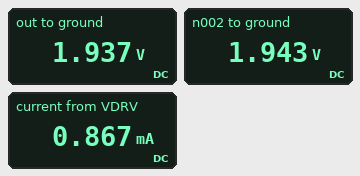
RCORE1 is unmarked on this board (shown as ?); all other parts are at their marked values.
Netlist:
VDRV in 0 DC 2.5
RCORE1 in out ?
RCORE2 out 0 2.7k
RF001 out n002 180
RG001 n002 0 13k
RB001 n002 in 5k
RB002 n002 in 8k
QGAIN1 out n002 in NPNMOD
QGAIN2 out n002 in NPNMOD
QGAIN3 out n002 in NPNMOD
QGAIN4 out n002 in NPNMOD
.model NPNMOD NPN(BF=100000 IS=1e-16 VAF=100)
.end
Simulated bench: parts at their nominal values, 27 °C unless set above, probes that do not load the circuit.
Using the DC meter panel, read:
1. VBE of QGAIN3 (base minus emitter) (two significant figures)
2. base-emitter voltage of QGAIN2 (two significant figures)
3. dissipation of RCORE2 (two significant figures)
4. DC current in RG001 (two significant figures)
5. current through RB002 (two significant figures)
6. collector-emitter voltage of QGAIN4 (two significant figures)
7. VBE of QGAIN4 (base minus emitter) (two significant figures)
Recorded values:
-560 mV
-560 mV
1.4 mW
150 µA
70 µA
-560 mV
-560 mV
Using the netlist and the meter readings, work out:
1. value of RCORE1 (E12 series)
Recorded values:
820 Ω
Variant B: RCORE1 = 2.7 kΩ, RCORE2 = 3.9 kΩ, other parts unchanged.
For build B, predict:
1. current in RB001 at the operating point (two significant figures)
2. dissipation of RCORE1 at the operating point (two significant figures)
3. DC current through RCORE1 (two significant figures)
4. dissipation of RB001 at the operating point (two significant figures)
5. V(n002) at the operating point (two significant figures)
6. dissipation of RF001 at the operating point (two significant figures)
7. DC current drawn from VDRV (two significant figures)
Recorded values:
160 µA
250 µW
300 µA
130 µW
1.7 V
2.9 µW
560 µA
